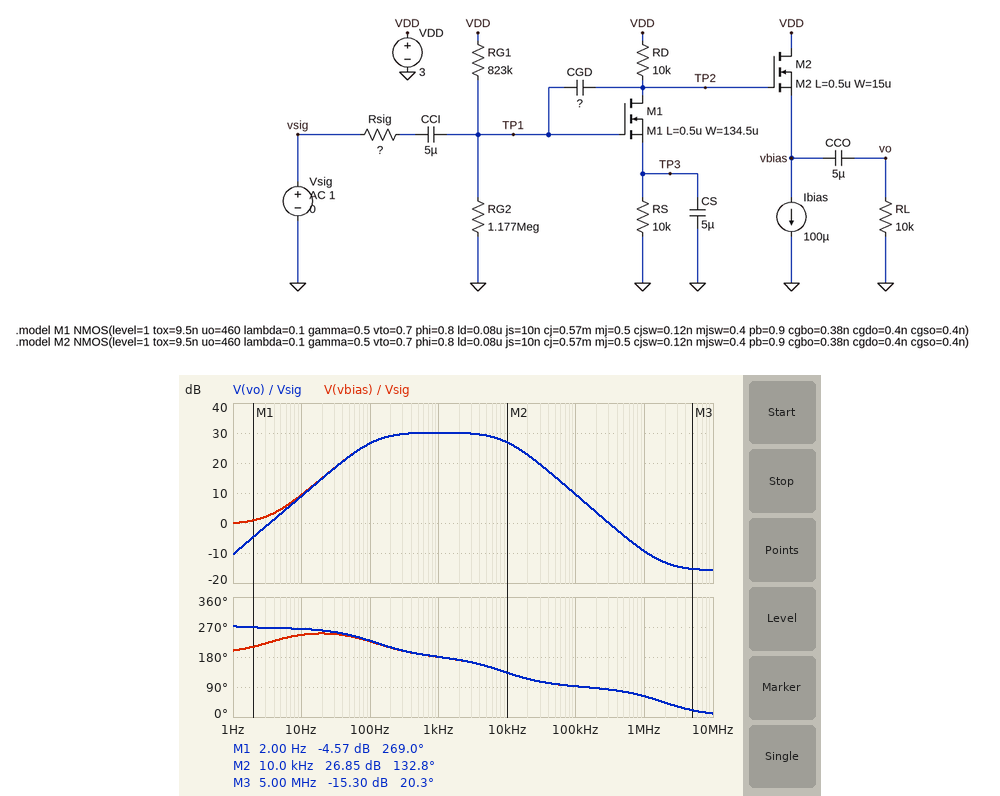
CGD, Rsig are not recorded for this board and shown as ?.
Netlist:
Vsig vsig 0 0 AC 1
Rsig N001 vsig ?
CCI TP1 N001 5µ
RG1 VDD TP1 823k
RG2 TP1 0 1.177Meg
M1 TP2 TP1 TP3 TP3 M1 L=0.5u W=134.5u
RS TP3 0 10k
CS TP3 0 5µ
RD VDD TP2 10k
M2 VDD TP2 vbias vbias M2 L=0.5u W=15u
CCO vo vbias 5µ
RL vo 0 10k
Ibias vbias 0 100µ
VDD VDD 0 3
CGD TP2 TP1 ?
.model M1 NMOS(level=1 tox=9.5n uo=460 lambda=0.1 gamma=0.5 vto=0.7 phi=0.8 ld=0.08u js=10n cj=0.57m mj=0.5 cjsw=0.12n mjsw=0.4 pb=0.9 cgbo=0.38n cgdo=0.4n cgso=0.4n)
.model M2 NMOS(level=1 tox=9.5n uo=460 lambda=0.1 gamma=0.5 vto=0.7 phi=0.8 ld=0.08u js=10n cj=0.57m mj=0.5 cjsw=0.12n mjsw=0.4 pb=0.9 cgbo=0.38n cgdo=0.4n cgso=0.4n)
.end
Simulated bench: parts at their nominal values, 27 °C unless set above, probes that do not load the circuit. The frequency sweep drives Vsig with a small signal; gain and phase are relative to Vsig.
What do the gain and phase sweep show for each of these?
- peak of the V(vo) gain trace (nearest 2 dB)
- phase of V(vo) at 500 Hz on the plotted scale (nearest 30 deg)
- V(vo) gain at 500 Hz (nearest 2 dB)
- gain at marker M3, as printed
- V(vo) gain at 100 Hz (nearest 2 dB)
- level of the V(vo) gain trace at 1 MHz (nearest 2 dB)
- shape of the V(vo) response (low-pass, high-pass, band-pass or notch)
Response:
30 dB
180 deg
30 dB
-15.30 dB
26 dB
-10 dB
band-pass
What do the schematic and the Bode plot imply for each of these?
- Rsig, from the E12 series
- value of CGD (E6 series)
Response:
1.2 kΩ
330 pF
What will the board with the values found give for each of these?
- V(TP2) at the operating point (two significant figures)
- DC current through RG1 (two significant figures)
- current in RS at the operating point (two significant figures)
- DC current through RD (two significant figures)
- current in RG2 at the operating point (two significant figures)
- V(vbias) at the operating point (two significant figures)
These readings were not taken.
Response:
2.0 V
1.5 µA
100 µA
100 µA
1.5 µA
1.1 V
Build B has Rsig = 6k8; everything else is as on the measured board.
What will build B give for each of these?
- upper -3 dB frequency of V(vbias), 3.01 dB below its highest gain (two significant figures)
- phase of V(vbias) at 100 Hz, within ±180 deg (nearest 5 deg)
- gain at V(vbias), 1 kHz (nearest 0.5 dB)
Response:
2.0 kHz
-135 deg
29.5 dB
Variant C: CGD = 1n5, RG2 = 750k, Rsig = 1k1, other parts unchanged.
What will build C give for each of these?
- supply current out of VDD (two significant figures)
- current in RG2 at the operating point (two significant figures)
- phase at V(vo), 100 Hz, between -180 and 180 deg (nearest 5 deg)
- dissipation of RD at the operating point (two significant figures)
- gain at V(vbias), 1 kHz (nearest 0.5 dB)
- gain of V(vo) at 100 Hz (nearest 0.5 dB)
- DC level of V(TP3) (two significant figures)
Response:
170 µA
1.9 µA
-135 deg
47 µW
28.5 dB
26.0 dB
690 mV
